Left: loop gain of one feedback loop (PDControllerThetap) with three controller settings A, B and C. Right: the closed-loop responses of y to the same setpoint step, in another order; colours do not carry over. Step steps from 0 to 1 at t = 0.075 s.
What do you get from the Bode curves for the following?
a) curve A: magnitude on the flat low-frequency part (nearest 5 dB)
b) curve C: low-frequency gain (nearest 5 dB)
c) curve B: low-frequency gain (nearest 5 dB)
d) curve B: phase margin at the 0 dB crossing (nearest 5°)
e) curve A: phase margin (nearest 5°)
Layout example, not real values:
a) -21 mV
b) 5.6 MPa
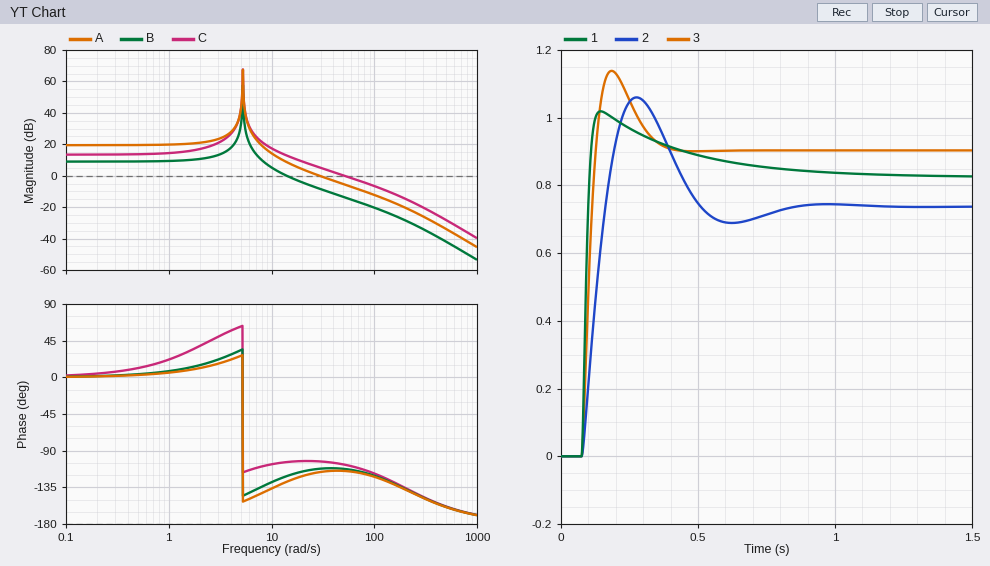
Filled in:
a) 20 dB
b) 15 dB
c) 10 dB
d) 60°
e) 65°
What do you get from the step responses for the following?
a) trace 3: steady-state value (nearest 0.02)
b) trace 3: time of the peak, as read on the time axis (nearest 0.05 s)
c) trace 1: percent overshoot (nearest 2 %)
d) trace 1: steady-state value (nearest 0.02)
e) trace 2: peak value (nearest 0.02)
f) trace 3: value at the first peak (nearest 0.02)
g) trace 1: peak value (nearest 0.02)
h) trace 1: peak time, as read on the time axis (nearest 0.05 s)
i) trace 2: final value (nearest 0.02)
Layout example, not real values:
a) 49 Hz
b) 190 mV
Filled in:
a) 0.90
b) 0.20 s
c) 24 %
d) 0.82
e) 1.06
f) 1.14
g) 1.02
h) 0.15 s
i) 0.74
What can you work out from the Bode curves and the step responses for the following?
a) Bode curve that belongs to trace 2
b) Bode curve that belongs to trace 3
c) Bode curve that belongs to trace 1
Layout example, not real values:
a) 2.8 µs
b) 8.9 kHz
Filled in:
a) B
b) A
c) C
